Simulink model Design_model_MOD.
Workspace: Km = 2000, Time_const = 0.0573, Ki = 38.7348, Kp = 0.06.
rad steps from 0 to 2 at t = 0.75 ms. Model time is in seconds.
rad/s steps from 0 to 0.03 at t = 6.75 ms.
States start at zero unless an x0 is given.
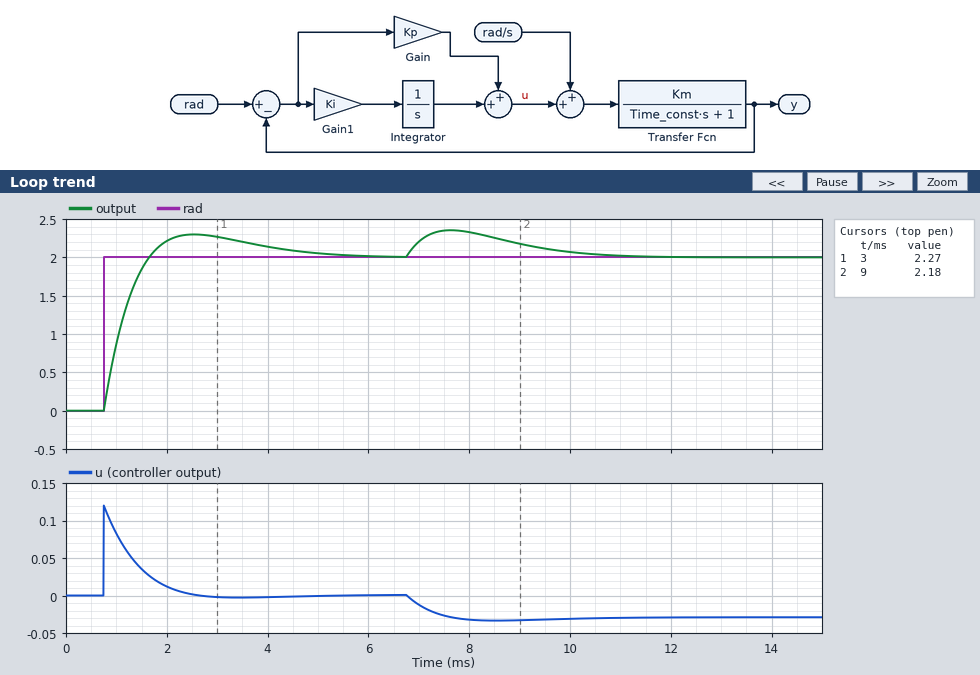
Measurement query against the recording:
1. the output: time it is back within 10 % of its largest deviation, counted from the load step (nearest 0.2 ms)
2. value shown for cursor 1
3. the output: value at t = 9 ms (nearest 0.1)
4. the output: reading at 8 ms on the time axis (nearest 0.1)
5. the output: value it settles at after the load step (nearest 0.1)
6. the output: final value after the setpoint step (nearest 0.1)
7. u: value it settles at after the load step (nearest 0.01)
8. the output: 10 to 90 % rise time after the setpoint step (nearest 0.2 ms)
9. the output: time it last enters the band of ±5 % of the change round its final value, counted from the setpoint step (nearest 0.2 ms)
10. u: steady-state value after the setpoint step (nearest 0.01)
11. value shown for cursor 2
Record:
3.8 ms
2.27
2.2
2.3
2.0
2.0
-0.03
0.6 ms
3.6 ms
0.00
2.18
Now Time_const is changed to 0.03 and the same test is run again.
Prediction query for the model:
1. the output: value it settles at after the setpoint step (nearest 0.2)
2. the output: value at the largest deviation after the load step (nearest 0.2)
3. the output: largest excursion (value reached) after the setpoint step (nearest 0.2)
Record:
2.0
2.4
2.2
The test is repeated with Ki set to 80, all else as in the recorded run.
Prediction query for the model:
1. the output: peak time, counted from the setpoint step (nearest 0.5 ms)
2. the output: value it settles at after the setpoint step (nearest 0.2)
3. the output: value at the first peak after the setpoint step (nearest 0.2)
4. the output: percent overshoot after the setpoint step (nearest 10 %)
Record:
1.5 ms
2.0
2.4
20 %
